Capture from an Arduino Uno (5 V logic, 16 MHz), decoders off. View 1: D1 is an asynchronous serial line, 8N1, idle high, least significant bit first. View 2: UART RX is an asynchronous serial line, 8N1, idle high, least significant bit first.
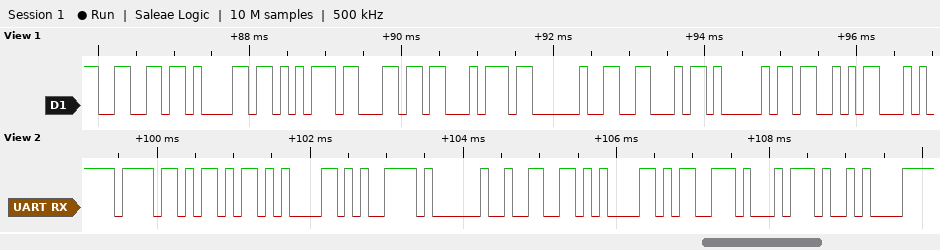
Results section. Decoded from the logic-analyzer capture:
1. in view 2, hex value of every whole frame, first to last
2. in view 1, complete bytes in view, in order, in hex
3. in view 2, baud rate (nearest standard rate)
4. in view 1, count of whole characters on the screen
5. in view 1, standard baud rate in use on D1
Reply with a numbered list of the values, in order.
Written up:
1. 6F 6B 61 79 20 66 61 73 74 0A
2. 66 61 75 6C 74 20 46 41 53
3. 9600 baud
4. 9
5. 9600 baud
